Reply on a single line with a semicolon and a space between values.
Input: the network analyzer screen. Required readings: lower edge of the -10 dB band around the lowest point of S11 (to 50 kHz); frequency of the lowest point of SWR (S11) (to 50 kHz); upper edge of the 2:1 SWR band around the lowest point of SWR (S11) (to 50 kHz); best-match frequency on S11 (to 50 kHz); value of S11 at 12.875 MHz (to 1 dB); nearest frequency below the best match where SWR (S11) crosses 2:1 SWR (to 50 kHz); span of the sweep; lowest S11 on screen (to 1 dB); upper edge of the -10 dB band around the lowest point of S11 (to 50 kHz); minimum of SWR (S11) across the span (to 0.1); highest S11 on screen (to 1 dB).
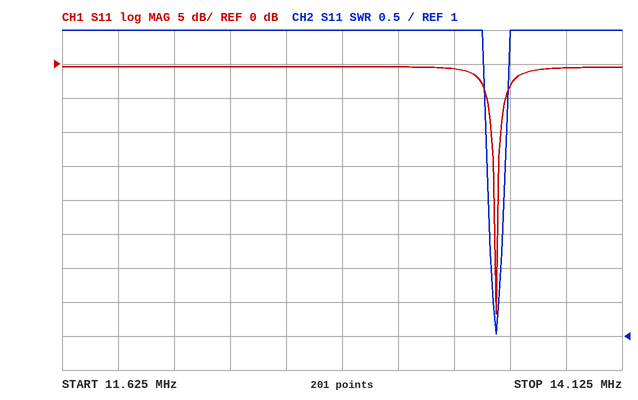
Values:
13.55 MHz; 13.55 MHz; 13.60 MHz; 13.55 MHz; 0 dB; 13.55 MHz; 2.5 MHz; -37 dB; 13.60 MHz; 1.0; 0 dB
